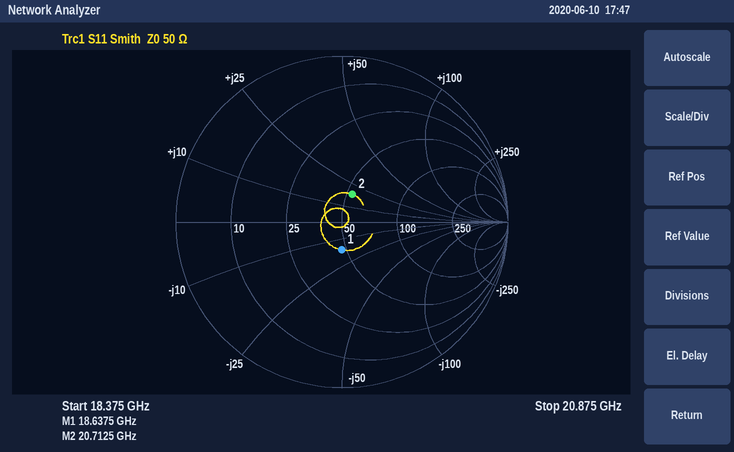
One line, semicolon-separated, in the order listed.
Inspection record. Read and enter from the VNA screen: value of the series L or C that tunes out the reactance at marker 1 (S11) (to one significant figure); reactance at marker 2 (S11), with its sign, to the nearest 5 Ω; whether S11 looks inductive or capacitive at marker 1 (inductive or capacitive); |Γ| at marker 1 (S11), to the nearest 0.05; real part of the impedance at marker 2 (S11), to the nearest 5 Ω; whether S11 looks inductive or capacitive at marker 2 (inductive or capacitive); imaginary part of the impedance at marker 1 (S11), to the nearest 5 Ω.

100 pH; +20 Ω; capacitive; 0.15; 55 Ω; inductive; -15 Ω
